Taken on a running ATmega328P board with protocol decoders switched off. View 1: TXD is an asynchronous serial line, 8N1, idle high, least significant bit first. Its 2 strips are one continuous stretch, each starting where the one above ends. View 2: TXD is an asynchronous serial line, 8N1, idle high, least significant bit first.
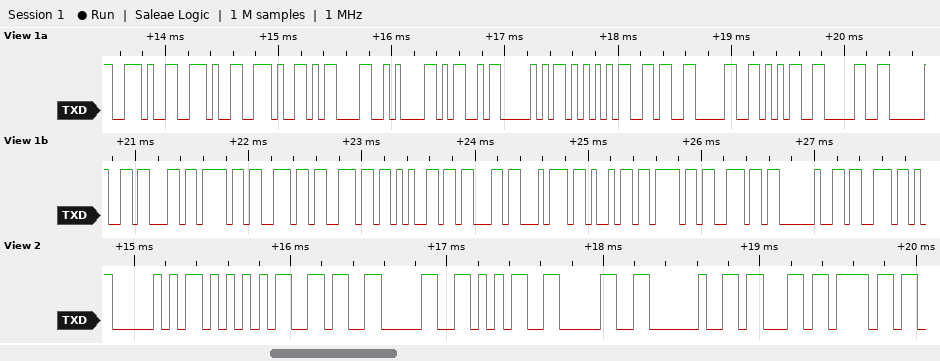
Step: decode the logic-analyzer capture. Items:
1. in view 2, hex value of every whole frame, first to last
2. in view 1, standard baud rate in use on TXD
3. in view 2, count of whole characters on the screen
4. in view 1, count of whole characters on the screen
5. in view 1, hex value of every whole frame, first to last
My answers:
0x50 0x55 0x36 0x30 0x35 0x30 0x20 0x63 0x6F
19200 baud
9
25
2E 2E 2E 0D 0A 4D 50 55 36 30 35 30 20 63 6F 6E 6E 65 63 74 69 6F 6E 20 73
